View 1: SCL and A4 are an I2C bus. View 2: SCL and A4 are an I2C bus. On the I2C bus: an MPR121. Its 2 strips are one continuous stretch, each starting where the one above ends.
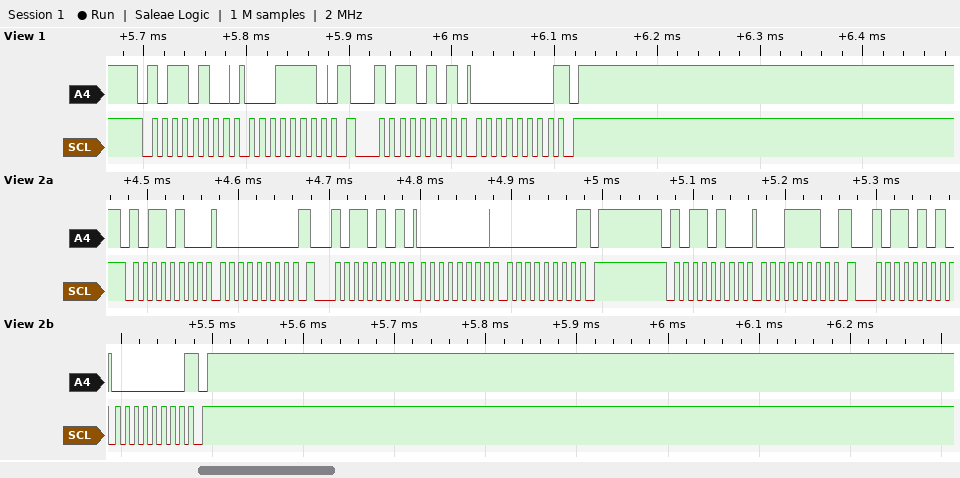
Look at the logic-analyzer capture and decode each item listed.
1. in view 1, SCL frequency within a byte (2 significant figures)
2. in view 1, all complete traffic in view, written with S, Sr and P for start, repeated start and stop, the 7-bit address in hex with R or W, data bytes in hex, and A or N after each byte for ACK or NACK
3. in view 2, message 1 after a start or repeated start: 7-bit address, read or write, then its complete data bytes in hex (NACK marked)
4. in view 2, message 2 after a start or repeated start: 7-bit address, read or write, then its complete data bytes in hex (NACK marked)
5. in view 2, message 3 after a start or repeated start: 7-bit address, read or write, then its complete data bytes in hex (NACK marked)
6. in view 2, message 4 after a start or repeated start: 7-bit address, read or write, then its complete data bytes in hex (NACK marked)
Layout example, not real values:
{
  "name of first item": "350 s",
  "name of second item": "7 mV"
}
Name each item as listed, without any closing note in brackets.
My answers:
{
  "in view 1, SCL frequency within a byte": "100 kHz",
  "in view 1, all complete traffic in view, written with S, Sr and P for start, repeated start and stop, the 7-bit address in hex with R or W, data bytes in hex, and A or N after each byte for ACK or NACK": "S 5AW A 1E A Sr 5AR A 00 N P",
  "in view 2, message 1 after a start or repeated start: 7-bit address, read or write, then its complete data bytes in hex": "0x5A write: 00",
  "in view 2, message 2 after a start or repeated start: 7-bit address, read or write, then its complete data bytes in hex": "0x5A read: 00 00 NACK",
  "in view 2, message 3 after a start or repeated start: 7-bit address, read or write, then its complete data bytes in hex": "0x5A write: 1E",
  "in view 2, message 4 after a start or repeated start: 7-bit address, read or write, then its complete data bytes in hex": "0x5A read: 00 NACK"
}
